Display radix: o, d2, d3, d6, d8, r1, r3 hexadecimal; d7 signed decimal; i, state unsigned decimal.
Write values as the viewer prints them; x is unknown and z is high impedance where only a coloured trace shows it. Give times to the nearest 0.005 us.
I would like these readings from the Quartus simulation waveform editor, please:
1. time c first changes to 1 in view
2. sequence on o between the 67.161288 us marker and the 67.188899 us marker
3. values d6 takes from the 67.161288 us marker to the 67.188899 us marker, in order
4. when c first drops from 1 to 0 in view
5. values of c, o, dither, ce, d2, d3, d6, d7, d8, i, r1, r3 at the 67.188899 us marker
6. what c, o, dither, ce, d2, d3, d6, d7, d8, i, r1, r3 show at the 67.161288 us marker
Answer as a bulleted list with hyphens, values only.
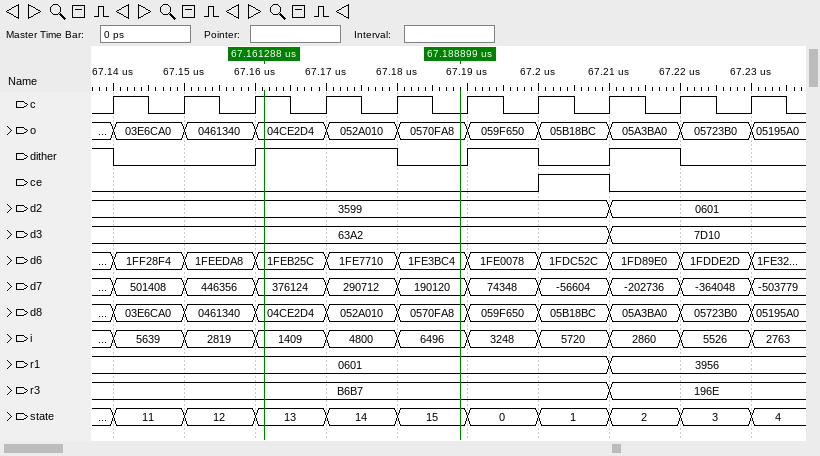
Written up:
- 67.14 us
- 04CE2D4, 052A010, 0570FA8
- 1FEB25C, 1FE7710, 1FE3BC4
- 67.145 us
- c=0, o=0570FA8, dither=0, ce=0, d2=3599, d3=63A2, d6=1FE3BC4, d7=190120, d8=0570FA8, i=6496, r1=0601, r3=B6B7
- c=1, o=04CE2D4, dither=1, ce=0, d2=3599, d3=63A2, d6=1FEB25C, d7=376124, d8=04CE2D4, i=1409, r1=0601, r3=B6B7
